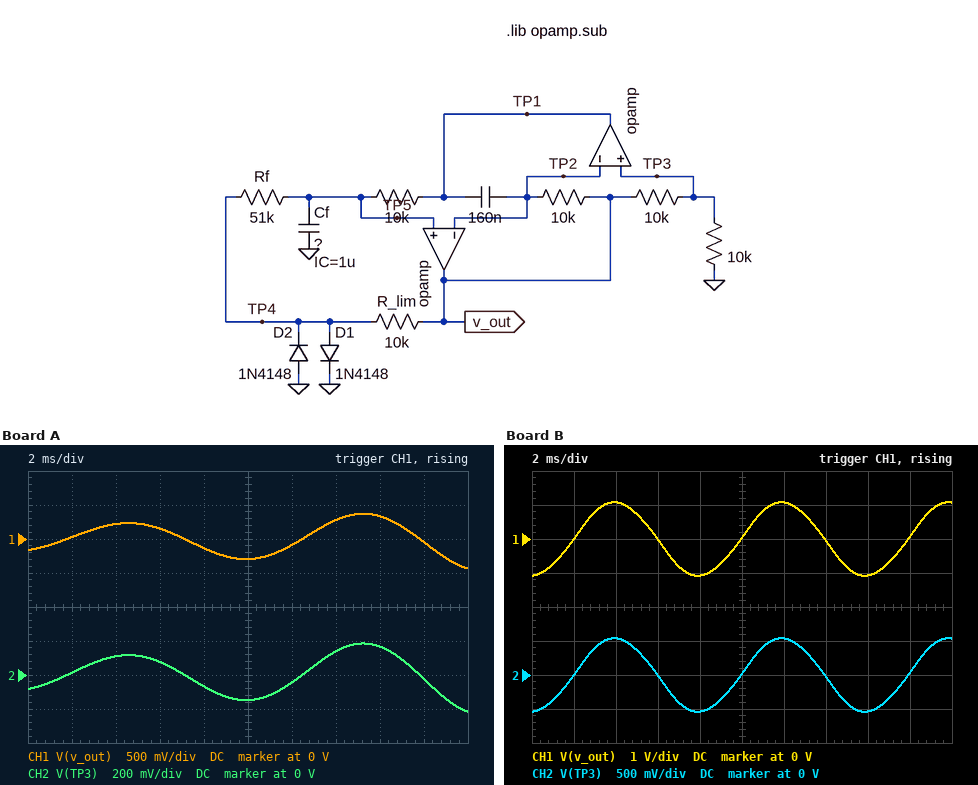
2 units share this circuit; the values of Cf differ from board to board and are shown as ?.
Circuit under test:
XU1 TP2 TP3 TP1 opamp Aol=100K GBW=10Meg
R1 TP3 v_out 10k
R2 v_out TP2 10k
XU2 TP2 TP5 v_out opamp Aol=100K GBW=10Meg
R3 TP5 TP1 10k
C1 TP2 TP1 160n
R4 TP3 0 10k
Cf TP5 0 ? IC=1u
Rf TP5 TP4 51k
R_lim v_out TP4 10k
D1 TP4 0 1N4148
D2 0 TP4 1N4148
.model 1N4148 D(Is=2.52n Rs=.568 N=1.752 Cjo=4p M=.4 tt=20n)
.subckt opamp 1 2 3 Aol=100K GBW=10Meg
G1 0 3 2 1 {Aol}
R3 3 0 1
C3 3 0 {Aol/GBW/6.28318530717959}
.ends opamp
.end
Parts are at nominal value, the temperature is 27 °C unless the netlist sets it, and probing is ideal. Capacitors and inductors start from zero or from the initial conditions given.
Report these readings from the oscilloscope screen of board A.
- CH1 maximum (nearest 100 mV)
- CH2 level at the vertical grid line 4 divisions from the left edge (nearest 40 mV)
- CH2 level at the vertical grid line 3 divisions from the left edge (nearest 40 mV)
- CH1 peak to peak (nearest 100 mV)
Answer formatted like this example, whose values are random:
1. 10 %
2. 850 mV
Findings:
1. 400 mV
2. -80 mV
3. 80 mV
4. 800 mV
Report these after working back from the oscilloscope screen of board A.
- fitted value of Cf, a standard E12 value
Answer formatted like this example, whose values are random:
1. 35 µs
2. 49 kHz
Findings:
1. 180 nF
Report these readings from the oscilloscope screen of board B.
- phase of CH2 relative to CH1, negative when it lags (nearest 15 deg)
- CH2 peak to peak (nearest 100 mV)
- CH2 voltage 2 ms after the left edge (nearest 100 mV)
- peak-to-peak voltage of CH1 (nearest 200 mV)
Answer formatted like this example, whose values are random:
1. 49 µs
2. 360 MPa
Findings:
1. 0 deg
2. 1.1 V
3. 0 V
4. 2.2 V
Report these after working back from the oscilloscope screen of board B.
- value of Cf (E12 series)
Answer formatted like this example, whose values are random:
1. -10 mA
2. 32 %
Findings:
1. 100 nF
